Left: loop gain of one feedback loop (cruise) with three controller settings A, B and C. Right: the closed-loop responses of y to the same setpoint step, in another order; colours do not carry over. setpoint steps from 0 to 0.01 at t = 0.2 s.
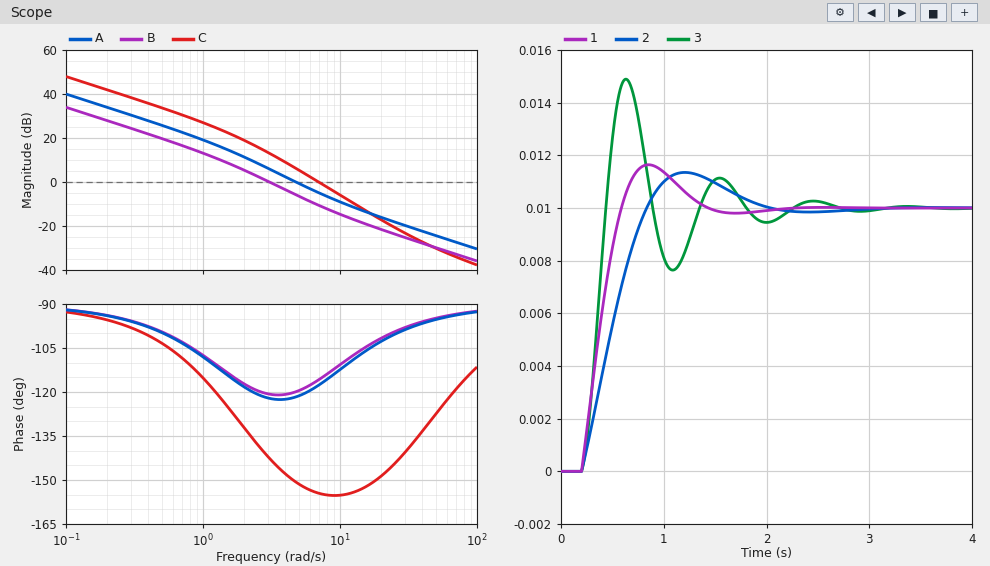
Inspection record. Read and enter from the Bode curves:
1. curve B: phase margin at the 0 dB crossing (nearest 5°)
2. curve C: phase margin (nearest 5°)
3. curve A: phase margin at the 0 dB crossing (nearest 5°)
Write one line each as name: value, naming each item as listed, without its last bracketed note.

curve B: phase margin at the 0 dB crossing: 60°
curve C: phase margin: 25°
curve A: phase margin at the 0 dB crossing: 60°
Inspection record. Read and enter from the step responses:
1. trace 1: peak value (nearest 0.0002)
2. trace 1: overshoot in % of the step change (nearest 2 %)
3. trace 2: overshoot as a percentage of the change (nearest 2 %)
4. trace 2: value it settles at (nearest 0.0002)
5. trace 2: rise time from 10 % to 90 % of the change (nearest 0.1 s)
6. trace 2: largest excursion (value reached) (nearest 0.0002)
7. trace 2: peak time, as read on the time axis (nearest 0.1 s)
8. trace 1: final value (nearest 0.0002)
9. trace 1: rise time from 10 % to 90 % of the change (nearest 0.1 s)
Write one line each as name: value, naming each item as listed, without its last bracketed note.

trace 1: peak value: 0.0116
trace 1: overshoot in % of the step change: 16 %
trace 2: overshoot as a percentage of the change: 14 %
trace 2: value it settles at: 0.0100
trace 2: rise time from 10 % to 90 % of the change: 0.5 s
trace 2: largest excursion (value reached): 0.0114
trace 2: peak time, as read on the time axis: 1.2 s
trace 1: final value: 0.0100
trace 1: rise time from 10 % to 90 % of the change: 0.3 s
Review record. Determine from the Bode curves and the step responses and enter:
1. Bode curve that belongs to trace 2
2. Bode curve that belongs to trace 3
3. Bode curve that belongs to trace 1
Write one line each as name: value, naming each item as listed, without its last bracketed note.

Bode curve that belongs to trace 2: B
Bode curve that belongs to trace 3: C
Bode curve that belongs to trace 1: A
